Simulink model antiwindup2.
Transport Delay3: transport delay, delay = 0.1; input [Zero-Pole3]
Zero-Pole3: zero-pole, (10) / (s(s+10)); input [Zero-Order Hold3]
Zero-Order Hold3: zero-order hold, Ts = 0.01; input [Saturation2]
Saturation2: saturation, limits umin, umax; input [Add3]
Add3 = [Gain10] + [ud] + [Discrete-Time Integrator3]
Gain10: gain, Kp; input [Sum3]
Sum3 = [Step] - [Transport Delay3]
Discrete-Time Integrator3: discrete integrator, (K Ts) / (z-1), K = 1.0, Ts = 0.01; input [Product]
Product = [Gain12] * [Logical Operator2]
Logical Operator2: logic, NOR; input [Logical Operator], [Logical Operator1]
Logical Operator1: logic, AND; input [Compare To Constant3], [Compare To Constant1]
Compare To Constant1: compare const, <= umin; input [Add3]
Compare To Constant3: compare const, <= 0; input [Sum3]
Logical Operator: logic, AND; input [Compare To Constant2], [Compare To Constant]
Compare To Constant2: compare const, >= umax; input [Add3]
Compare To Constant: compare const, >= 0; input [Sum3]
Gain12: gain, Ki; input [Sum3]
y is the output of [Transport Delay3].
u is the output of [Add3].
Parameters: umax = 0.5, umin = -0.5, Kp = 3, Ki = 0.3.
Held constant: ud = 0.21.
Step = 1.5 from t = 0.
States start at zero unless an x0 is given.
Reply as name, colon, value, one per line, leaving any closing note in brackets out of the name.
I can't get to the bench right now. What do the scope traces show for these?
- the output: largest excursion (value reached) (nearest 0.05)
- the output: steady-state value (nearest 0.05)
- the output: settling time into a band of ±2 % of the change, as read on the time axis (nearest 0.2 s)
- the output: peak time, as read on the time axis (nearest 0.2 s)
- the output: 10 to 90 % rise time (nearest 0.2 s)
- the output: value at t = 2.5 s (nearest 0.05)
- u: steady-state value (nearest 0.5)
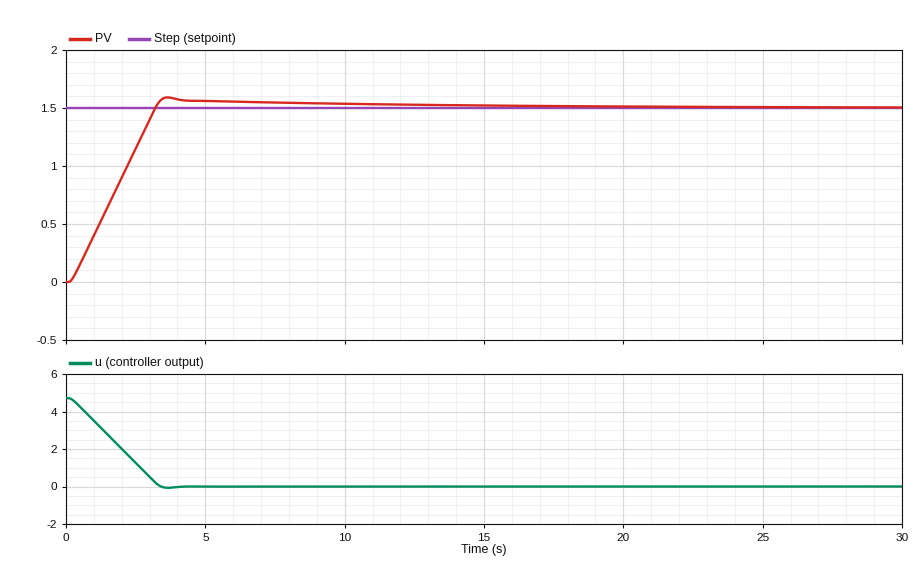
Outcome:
the output: largest excursion (value reached): 1.60
the output: steady-state value: 1.50
the output: settling time into a band of ±2 % of the change, as read on the time axis: 11.8 s
the output: peak time, as read on the time axis: 3.6 s
the output: 10 to 90 % rise time: 2.4 s
the output: value at t = 2.5 s: 1.15
u: steady-state value: 0.0
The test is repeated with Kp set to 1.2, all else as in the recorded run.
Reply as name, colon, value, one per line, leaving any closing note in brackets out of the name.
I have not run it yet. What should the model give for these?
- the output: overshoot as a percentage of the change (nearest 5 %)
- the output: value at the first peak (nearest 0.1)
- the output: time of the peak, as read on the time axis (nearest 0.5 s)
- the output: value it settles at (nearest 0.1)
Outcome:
the output: overshoot as a percentage of the change: 10 %
the output: value at the first peak: 1.7
the output: time of the peak, as read on the time axis: 4.5 s
the output: value it settles at: 1.5
